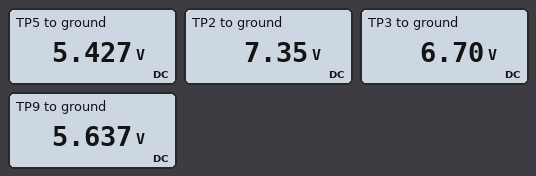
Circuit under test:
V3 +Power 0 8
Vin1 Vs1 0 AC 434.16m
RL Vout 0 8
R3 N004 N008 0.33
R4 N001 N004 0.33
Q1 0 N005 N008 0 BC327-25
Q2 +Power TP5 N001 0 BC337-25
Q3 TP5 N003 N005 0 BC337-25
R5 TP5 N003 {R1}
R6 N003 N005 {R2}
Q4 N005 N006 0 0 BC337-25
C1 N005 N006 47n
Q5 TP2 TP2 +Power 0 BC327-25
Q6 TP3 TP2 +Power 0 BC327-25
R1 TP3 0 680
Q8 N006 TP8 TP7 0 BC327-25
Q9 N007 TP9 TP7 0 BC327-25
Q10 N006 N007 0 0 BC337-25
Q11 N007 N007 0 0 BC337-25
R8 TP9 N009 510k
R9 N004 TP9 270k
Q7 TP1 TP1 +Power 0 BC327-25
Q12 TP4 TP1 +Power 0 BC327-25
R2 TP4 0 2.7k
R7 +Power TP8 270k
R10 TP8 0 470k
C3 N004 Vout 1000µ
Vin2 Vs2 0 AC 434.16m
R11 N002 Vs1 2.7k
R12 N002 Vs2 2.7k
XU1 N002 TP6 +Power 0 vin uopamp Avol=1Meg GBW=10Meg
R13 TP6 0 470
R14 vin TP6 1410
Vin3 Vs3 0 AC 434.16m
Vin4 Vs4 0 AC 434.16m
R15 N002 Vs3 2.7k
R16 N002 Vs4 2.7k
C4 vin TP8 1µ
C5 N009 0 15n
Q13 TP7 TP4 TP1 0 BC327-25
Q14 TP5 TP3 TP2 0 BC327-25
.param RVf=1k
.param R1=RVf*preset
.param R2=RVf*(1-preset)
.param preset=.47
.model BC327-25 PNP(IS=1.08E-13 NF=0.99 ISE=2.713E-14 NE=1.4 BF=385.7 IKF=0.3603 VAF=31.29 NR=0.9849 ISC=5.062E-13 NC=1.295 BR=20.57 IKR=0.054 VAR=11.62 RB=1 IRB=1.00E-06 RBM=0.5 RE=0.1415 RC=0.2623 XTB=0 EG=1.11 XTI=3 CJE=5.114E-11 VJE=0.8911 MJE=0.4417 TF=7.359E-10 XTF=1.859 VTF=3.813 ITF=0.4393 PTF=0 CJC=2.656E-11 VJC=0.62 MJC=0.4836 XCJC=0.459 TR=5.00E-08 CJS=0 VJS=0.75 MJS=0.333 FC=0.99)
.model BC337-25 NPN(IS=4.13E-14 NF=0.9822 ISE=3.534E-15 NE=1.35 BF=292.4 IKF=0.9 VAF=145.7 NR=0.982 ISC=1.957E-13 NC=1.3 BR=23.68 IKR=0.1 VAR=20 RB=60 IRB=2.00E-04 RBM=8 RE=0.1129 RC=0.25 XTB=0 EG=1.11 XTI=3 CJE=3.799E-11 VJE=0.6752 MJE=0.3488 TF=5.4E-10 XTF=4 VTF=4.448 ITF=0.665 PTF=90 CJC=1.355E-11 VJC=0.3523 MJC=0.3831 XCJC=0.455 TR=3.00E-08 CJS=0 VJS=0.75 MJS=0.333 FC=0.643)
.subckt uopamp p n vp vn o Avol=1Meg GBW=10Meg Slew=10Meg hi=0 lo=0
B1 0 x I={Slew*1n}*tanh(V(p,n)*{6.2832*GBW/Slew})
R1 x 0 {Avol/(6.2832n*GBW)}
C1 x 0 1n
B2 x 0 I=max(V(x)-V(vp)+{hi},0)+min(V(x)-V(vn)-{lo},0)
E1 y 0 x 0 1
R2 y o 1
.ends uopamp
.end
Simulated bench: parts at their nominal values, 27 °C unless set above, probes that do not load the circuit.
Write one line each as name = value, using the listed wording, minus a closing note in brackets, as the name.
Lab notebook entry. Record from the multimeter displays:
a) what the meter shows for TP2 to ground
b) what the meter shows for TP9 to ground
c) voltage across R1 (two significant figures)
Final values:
what the meter shows for TP2 to ground = 7.35 V
what the meter shows for TP9 to ground = 5.637 V
voltage across R1 = 6.7 V
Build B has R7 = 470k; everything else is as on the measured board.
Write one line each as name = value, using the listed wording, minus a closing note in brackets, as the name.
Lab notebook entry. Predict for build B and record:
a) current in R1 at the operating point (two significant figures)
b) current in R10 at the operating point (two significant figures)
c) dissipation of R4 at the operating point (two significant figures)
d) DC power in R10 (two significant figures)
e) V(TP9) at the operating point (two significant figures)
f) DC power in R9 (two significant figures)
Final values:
current in R1 at the operating point = 9.9 mA
current in R10 at the operating point = 10 µA
dissipation of R4 at the operating point = 5.1 µW
DC power in R10 = 49 µW
V(TP9) at the operating point = 4.8 V
DC power in R9 = 2.8 µW
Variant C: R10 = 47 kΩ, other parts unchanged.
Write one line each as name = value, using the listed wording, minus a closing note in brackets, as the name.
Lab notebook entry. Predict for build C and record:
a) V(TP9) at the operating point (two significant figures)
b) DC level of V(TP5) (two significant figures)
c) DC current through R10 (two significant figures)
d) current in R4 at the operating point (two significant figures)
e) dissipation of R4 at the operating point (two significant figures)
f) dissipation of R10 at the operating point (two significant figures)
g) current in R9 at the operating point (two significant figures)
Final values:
V(TP9) at the operating point = 1.4 V
DC level of V(TP5) = 1.3 V
DC current through R10 = 29 µA
current in R4 at the operating point = 3.8 mA
dissipation of R4 at the operating point = 4.8 µW
dissipation of R10 at the operating point = 40 µW
current in R9 at the operating point = 2.7 µA
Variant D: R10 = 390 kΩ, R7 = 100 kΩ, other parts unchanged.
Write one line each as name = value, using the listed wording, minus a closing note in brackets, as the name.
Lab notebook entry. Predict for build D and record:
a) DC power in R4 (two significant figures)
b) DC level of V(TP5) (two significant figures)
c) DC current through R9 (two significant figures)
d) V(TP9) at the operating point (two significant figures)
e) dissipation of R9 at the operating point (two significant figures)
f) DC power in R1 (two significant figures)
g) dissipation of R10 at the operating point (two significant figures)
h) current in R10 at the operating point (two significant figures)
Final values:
DC power in R4 = 5.3 µW
DC level of V(TP5) = 6.4 V
DC current through R9 = 3.1 µA
V(TP9) at the operating point = 6.6 V
dissipation of R9 at the operating point = 2.6 µW
DC power in R1 = 66 mW
dissipation of R10 at the operating point = 110 µW
current in R10 at the operating point = 17 µA
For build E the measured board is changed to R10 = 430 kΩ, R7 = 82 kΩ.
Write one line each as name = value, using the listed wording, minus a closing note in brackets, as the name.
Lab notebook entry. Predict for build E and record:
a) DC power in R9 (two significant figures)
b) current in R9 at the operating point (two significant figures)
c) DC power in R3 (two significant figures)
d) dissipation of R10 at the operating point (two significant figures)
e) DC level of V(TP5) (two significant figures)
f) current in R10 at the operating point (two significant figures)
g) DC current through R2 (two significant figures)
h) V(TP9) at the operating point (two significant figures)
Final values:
DC power in R9 = 500 nW
current in R9 at the operating point = 1.4 µA
DC power in R3 = 5.4 µW
dissipation of R10 at the operating point = 110 µW
DC level of V(TP5) = 7.1 V
current in R10 at the operating point = 16 µA
DC current through R2 = 2.5 mA
V(TP9) at the operating point = 6.8 V
